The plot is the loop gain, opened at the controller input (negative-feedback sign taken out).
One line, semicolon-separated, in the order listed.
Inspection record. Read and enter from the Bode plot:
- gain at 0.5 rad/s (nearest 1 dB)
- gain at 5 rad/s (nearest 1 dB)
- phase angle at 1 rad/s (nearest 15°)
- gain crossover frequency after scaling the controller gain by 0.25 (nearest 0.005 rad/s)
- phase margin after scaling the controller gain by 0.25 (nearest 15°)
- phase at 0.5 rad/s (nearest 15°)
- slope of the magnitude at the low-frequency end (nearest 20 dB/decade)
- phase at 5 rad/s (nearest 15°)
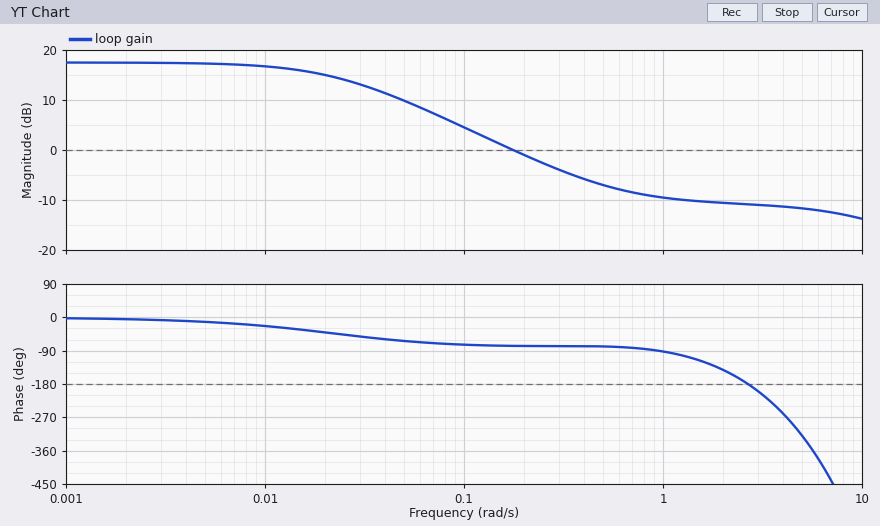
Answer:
-7 dB; -12 dB; -90°; 0.035 rad/s; 120°; -75°; 0 dB/decade; -315°
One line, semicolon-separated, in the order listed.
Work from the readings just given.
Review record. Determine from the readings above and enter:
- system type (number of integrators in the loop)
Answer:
0
